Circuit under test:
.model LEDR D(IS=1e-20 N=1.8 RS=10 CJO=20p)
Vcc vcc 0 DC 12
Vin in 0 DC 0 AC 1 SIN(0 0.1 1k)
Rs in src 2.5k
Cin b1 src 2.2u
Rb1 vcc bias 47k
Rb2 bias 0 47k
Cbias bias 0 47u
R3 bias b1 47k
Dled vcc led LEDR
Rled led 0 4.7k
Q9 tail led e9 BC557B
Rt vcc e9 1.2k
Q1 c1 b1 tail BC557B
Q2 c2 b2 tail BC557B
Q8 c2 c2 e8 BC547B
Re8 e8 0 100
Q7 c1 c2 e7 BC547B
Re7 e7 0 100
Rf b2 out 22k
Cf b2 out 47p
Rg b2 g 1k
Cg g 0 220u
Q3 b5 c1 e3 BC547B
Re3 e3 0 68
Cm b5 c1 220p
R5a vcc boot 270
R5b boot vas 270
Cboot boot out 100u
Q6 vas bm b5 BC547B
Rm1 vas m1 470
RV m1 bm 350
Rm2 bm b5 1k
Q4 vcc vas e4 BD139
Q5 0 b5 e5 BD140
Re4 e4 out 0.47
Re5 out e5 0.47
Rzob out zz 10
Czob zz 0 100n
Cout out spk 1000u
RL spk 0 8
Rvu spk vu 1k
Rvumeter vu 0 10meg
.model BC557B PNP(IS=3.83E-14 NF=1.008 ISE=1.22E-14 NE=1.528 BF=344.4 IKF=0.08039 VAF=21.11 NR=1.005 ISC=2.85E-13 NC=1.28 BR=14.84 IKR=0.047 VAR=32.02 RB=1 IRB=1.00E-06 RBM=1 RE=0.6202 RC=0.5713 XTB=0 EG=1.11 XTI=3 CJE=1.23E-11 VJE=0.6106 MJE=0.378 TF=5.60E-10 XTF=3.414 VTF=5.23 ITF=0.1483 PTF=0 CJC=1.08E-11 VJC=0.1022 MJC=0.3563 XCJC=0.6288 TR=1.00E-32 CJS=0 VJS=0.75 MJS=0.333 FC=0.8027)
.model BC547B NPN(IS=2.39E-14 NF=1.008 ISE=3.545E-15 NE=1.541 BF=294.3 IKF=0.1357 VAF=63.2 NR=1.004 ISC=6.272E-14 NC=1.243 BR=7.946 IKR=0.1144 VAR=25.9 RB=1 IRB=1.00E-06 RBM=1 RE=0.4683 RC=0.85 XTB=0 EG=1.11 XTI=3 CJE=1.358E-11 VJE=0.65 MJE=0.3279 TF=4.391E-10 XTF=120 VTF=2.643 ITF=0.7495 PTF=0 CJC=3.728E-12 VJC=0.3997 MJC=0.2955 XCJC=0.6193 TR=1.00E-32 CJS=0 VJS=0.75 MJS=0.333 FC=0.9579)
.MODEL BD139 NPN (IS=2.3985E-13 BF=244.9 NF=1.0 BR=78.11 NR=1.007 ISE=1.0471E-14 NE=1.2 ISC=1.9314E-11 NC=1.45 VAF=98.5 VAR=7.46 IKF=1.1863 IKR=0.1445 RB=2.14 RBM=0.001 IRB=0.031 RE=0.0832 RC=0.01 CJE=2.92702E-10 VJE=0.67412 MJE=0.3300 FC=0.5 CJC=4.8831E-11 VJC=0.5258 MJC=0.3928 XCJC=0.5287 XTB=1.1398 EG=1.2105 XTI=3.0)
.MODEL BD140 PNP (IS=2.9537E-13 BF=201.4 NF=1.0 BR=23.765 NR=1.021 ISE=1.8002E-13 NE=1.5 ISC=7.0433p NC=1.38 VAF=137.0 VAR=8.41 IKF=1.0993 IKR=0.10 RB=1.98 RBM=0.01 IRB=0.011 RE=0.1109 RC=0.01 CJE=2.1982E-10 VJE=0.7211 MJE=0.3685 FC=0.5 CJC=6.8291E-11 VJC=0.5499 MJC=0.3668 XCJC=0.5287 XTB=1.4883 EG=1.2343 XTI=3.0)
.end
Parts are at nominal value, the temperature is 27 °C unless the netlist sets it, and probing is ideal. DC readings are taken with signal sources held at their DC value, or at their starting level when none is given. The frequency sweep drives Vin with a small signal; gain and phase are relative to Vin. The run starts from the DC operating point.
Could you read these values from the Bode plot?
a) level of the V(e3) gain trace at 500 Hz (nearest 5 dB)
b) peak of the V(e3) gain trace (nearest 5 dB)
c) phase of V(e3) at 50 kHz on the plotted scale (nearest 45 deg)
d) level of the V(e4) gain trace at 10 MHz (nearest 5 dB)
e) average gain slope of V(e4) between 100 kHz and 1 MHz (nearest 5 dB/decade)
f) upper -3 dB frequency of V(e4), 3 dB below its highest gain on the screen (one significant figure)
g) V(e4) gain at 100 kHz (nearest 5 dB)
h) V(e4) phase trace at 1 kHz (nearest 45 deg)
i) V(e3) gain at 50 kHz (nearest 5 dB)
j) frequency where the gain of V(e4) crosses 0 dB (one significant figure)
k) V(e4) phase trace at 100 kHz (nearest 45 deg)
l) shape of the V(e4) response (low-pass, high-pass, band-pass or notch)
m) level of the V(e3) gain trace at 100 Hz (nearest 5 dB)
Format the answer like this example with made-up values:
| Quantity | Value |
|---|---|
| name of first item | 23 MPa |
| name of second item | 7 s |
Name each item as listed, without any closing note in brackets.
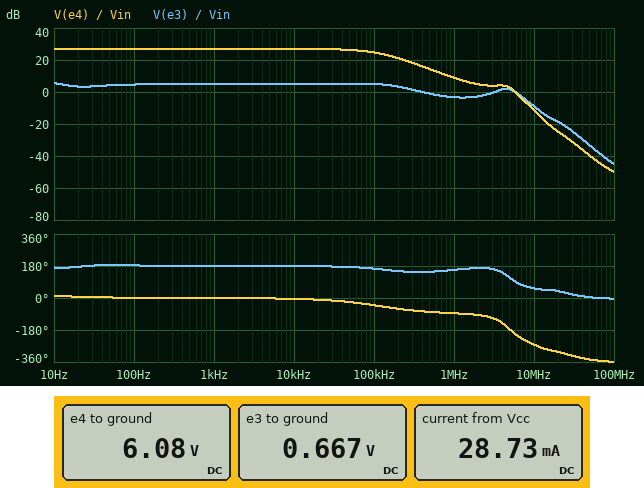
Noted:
| Quantity | Value |
|---|---|
| level of the V(e3) gain trace at 500 Hz | 5 dB |
| peak of the V(e3) gain trace | 5 dB |
| phase of V(e3) at 50 kHz on the plotted scale | 180 deg |
| level of the V(e4) gain trace at 10 MHz | -10 dB |
| average gain slope of V(e4) between 100 kHz and 1 MHz | -15 dB/decade |
| upper -3 dB frequency of V(e4), 3 dB below its highest gain on the screen | 100 kHz |
| V(e4) gain at 100 kHz | 25 dB |
| V(e4) phase trace at 1 kHz | 0 deg |
| V(e3) gain at 50 kHz | 5 dB |
| frequency where the gain of V(e4) crosses 0 dB | 6 MHz |
| V(e4) phase trace at 100 kHz | -45 deg |
| shape of the V(e4) response | low-pass |
| level of the V(e3) gain trace at 100 Hz | 5 dB |
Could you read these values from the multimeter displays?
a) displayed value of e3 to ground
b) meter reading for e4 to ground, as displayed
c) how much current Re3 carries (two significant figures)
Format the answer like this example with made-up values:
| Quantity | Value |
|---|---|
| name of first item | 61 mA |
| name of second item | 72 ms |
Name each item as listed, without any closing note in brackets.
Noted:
| Quantity | Value |
|---|---|
| displayed value of e3 to ground | 0.667 V |
| meter reading for e4 to ground, as displayed | 6.08 V |
| how much current Re3 carries | 9.8 mA |
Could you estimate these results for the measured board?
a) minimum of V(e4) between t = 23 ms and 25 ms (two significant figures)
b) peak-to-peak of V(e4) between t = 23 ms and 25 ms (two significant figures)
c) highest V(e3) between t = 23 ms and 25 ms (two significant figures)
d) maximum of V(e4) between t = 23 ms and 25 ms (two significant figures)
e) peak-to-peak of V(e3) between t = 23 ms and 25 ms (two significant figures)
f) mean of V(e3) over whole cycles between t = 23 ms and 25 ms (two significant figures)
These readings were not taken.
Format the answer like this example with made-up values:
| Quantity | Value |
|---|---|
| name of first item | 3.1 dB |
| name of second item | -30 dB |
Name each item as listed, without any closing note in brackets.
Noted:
| Quantity | Value |
|---|---|
| minimum of V(e4) between t = 23 ms and 25 ms | 3.9 V |
| peak-to-peak of V(e4) between t = 23 ms and 25 ms | 4.5 V |
| highest V(e3) between t = 23 ms and 25 ms | 850 mV |
| maximum of V(e4) between t = 23 ms and 25 ms | 8.4 V |
| peak-to-peak of V(e3) between t = 23 ms and 25 ms | 360 mV |
| mean of V(e3) over whole cycles between t = 23 ms and 25 ms | 670 mV |
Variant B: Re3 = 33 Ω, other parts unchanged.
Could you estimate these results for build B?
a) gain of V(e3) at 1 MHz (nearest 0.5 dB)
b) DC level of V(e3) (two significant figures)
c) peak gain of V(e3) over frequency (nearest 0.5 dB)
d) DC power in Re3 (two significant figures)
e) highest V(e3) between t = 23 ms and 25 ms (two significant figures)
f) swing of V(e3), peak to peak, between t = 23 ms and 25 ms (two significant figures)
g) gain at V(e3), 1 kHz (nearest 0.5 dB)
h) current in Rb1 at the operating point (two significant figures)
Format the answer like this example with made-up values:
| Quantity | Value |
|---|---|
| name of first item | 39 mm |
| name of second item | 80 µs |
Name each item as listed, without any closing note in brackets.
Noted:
| Quantity | Value |
|---|---|
| gain of V(e3) at 1 MHz | -9.5 dB |
| DC level of V(e3) | 320 mV |
| peak gain of V(e3) over frequency | 1.0 dB |
| DC power in Re3 | 3.2 mW |
| highest V(e3) between t = 23 ms and 25 ms | 410 mV |
| swing of V(e3), peak to peak, between t = 23 ms and 25 ms | 170 mV |
| gain at V(e3), 1 kHz | -1.5 dB |
| current in Rb1 at the operating point | 130 µA |
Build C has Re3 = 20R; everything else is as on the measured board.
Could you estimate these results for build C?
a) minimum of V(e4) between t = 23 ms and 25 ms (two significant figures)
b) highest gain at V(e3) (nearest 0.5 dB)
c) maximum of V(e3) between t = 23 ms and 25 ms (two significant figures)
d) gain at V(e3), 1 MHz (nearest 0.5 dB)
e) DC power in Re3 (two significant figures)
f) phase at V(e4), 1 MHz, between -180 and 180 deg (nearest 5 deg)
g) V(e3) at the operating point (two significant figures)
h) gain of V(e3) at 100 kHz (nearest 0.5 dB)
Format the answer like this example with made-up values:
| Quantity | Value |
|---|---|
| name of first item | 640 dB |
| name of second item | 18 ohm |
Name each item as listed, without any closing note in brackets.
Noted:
| Quantity | Value |
|---|---|
| minimum of V(e4) between t = 23 ms and 25 ms | 3.9 V |
| highest gain at V(e3) | -3.5 dB |
| maximum of V(e3) between t = 23 ms and 25 ms | 250 mV |
| gain at V(e3), 1 MHz | -14.0 dB |
| DC power in Re3 | 1.9 mW |
| phase at V(e4), 1 MHz, between -180 and 180 deg | -80 deg |
| V(e3) at the operating point | 200 mV |
| gain of V(e3) at 100 kHz | -5.5 dB |
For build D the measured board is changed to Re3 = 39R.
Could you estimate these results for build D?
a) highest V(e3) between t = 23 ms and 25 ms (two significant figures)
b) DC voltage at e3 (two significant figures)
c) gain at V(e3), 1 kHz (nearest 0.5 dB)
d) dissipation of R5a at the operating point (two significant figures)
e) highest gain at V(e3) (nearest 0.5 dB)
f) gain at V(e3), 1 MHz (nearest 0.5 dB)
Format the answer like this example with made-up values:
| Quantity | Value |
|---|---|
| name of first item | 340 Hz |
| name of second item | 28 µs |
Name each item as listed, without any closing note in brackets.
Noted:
| Quantity | Value |
|---|---|
| highest V(e3) between t = 23 ms and 25 ms | 490 mV |
| DC voltage at e3 | 380 mV |
| gain at V(e3), 1 kHz | 0 dB |
| dissipation of R5a at the operating point | 26 mW |
| highest gain at V(e3) | 2.5 dB |
| gain at V(e3), 1 MHz | -8.0 dB |
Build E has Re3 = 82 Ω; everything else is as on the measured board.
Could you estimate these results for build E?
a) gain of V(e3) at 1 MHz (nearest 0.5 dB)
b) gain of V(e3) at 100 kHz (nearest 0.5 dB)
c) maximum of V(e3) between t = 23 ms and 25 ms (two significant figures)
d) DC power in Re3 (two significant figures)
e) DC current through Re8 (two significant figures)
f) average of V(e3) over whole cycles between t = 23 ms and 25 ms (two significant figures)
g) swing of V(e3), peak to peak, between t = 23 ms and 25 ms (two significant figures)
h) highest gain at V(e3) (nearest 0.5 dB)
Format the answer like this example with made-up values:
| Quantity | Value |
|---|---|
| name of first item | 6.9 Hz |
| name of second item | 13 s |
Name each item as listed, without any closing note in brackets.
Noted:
| Quantity | Value |
|---|---|
| gain of V(e3) at 1 MHz | -1.5 dB |
| gain of V(e3) at 100 kHz | 6.5 dB |
| maximum of V(e3) between t = 23 ms and 25 ms | 1.0 V |
| DC power in Re3 | 7.9 mW |
| DC current through Re8 | 500 µA |
| average of V(e3) over whole cycles between t = 23 ms and 25 ms | 810 mV |
| swing of V(e3), peak to peak, between t = 23 ms and 25 ms | 430 mV |
| highest gain at V(e3) | 9.0 dB |
